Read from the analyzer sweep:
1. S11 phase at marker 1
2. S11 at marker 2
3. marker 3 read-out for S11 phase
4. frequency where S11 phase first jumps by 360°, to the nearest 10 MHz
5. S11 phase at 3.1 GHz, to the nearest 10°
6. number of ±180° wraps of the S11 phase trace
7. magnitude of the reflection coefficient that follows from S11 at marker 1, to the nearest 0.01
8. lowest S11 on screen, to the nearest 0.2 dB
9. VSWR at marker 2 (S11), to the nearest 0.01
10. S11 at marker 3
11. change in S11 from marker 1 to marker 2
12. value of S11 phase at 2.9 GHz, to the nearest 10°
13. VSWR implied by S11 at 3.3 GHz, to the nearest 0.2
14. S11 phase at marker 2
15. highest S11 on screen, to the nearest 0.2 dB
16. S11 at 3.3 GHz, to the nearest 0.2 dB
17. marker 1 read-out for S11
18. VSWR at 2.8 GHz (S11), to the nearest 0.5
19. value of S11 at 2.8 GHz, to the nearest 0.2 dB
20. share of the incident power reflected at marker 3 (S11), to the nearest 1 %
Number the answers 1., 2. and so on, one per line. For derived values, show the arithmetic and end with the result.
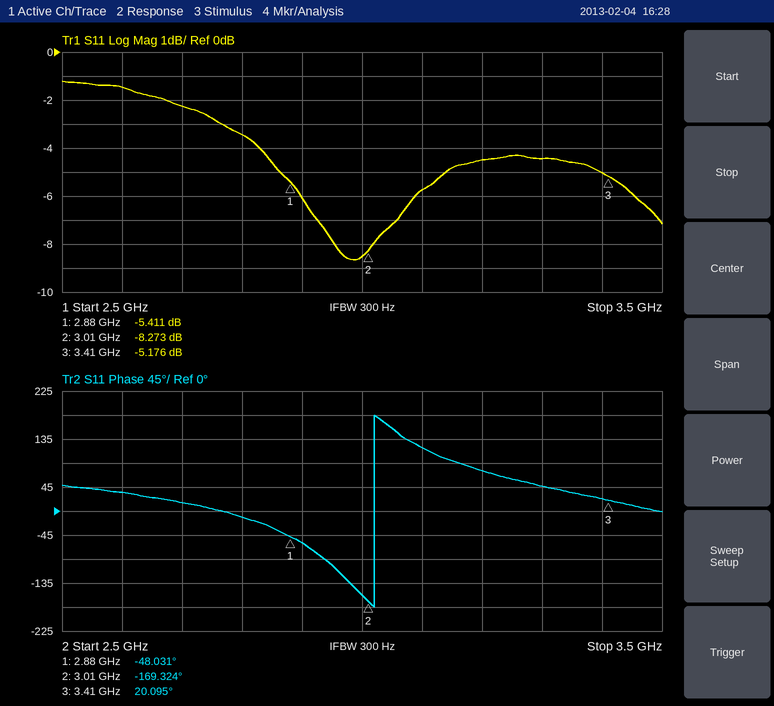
1. -48.031°
2. -8.273 dB
3. 20.095°
4. 3.02 GHz
5. 120°
6. 1
7. 10^(-5.411/20) ≈ 0.54
8. -8.6 dB
9. (1 + 0.3858)/(1 − 0.3858) ≈ 2.26
10. -5.176 dB
11. -8.273 − (-5.411) = -2.862 dB
12. -60°
13. |Γ| = 10^(-4.4/20) = 0.6026; VSWR = (1 + 0.6026)/(1 − 0.6026) ≈ 4.0
14. -169.324°
15. -1.2 dB
16. -4.4 dB
17. -5.411 dB
18. |Γ| = 10^(-3.4/20) = 0.6761; VSWR = (1 + 0.6761)/(1 − 0.6761) ≈ 5.17, so 5.0 to the nearest 0.5
19. -3.4 dB
20. 10^(-5.176/10) ≈ 30 %
